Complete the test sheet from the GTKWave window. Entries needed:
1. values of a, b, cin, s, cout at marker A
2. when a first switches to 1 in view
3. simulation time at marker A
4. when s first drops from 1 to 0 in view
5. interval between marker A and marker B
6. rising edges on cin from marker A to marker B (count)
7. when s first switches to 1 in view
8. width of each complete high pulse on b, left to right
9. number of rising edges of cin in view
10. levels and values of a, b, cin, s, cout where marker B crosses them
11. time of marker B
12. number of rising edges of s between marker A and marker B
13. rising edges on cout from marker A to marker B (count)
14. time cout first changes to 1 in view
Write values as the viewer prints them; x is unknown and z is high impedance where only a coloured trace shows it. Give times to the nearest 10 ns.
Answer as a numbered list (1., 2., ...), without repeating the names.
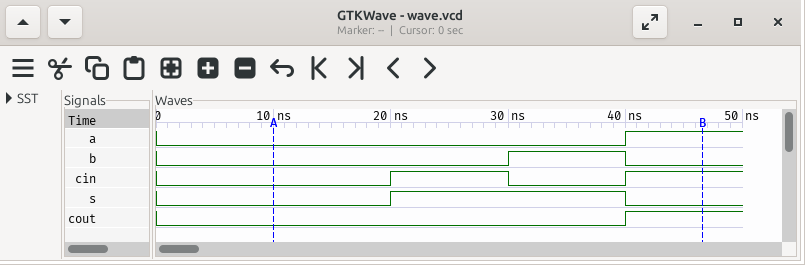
1. a=0, b=0, cin=0, s=0, cout=0
2. 40 ns
3. 10 ns
4. 40 ns
5. 40 ns
6. 2
7. 20 ns
8. 10 ns
9. 2
10. a=1, b=0, cin=1, s=0, cout=1
11. 50 ns
12. 1
13. 1
14. 40 ns
